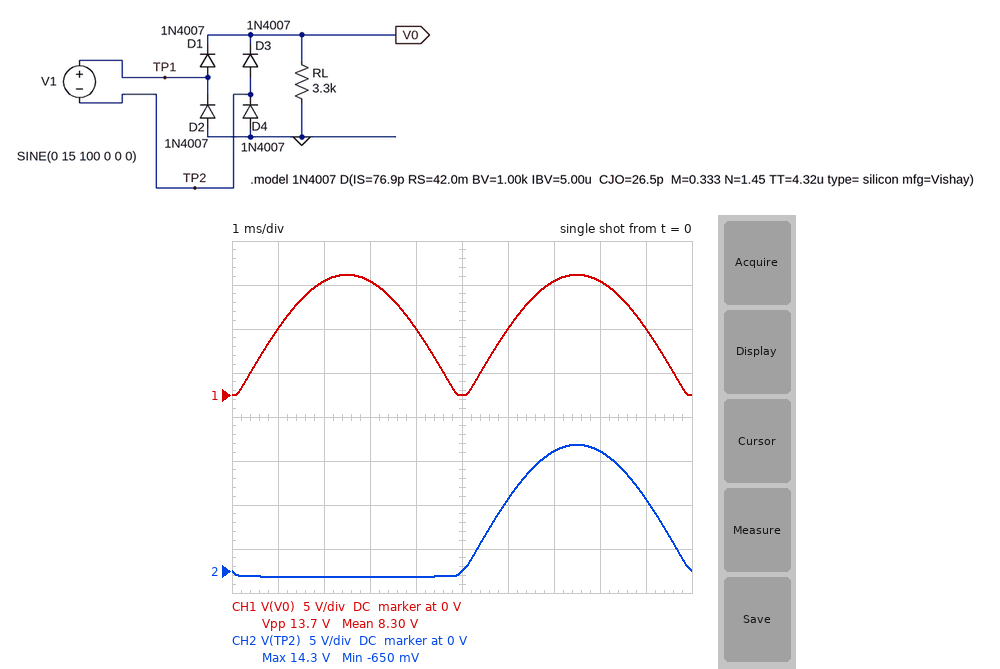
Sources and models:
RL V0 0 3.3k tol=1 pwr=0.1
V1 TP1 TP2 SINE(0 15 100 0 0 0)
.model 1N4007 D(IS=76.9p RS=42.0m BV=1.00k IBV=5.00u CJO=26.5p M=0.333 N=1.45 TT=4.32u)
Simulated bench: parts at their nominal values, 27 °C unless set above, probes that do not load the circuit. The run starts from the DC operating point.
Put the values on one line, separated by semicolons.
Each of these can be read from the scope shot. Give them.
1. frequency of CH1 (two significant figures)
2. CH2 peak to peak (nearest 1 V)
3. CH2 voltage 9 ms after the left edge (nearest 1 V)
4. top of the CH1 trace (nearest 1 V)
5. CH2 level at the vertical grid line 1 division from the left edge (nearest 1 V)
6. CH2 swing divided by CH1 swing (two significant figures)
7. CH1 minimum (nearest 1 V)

200 Hz; 15 V; 8 V; 14 V; -1 V; 1.1; 0 V
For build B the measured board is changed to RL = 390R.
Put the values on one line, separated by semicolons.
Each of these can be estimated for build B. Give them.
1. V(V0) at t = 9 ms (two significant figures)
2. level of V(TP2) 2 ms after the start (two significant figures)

7.4 V; -750 mV
